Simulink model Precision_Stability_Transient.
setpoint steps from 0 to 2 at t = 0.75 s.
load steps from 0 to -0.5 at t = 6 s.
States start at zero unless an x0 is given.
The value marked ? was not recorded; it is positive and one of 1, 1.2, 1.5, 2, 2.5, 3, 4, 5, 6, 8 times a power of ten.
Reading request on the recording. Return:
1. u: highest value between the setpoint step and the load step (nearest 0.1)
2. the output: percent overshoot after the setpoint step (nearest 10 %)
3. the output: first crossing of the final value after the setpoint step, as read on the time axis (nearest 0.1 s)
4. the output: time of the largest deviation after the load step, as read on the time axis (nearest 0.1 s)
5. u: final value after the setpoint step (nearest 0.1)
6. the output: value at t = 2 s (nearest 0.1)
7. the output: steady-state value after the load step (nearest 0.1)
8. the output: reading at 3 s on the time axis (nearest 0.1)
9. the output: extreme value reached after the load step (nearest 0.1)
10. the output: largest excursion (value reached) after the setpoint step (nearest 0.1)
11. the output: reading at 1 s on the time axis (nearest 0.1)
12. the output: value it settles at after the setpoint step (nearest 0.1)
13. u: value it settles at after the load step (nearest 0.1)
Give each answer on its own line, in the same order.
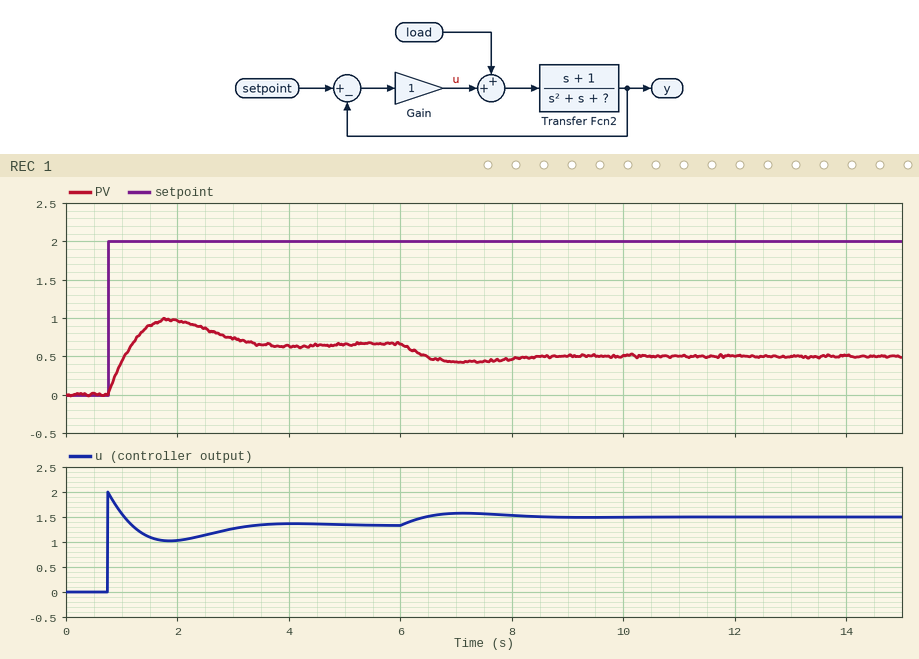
2.0
50 %
1.2 s
7.1 s
1.3
1.0
0.5
0.7
0.4
1.0
0.4
0.7
1.5
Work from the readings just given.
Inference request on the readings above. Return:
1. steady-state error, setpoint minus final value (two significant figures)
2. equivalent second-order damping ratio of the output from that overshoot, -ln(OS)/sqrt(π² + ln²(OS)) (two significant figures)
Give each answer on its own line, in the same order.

1.3
0.22
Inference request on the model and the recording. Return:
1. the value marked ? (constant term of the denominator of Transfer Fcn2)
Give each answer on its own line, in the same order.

2
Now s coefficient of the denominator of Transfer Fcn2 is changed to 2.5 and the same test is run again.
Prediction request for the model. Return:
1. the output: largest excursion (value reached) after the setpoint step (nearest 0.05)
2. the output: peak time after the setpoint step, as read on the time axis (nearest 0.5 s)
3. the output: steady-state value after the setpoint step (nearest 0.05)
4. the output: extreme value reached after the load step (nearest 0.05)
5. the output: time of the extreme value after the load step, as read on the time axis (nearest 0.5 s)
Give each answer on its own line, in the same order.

0.70
2.0 s
0.65
0.50
7.5 s
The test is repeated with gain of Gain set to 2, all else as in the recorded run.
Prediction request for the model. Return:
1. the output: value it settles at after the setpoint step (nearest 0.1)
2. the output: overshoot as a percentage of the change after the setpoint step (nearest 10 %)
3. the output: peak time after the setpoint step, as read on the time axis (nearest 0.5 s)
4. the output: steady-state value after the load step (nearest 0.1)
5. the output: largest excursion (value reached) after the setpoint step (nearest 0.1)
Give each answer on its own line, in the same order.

1.0
40 %
1.5 s
0.9
1.4
